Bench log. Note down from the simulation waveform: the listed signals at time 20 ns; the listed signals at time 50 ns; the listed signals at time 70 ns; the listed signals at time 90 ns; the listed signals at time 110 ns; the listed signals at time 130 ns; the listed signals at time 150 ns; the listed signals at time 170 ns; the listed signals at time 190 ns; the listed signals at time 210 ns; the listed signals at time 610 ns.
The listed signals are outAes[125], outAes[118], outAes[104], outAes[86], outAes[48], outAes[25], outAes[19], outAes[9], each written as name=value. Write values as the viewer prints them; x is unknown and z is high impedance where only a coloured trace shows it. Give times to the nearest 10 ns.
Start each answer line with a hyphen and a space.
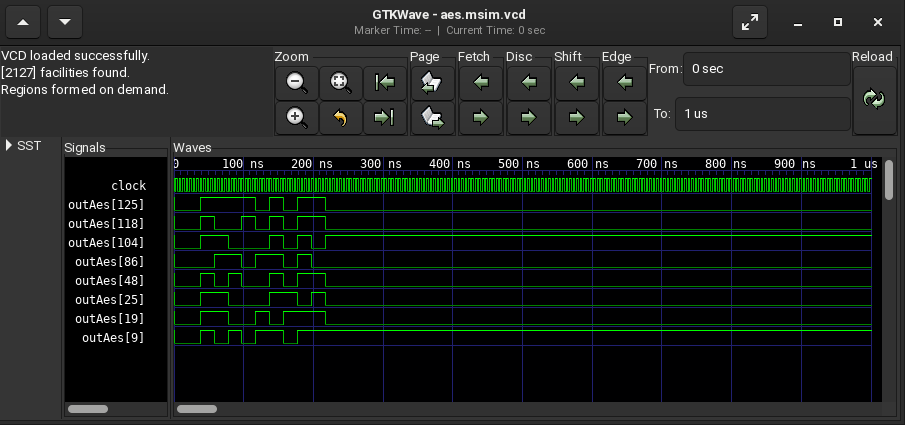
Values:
- outAes[125]=0, outAes[118]=0, outAes[104]=0, outAes[86]=0, outAes[48]=0, outAes[25]=0, outAes[19]=0, outAes[9]=0
- outAes[125]=1, outAes[118]=1, outAes[104]=1, outAes[86]=0, outAes[48]=1, outAes[25]=1, outAes[19]=1, outAes[9]=1
- outAes[125]=1, outAes[118]=0, outAes[104]=1, outAes[86]=1, outAes[48]=0, outAes[25]=1, outAes[19]=1, outAes[9]=0
- outAes[125]=1, outAes[118]=0, outAes[104]=0, outAes[86]=1, outAes[48]=1, outAes[25]=0, outAes[19]=0, outAes[9]=1
- outAes[125]=1, outAes[118]=1, outAes[104]=0, outAes[86]=0, outAes[48]=0, outAes[25]=0, outAes[19]=0, outAes[9]=0
- outAes[125]=0, outAes[118]=0, outAes[104]=0, outAes[86]=1, outAes[48]=0, outAes[25]=0, outAes[19]=1, outAes[9]=1
- outAes[125]=1, outAes[118]=1, outAes[104]=1, outAes[86]=1, outAes[48]=1, outAes[25]=1, outAes[19]=0, outAes[9]=1
- outAes[125]=0, outAes[118]=0, outAes[104]=0, outAes[86]=0, outAes[48]=0, outAes[25]=1, outAes[19]=1, outAes[9]=0
- outAes[125]=1, outAes[118]=1, outAes[104]=1, outAes[86]=1, outAes[48]=1, outAes[25]=0, outAes[19]=1, outAes[9]=1
- outAes[125]=1, outAes[118]=1, outAes[104]=0, outAes[86]=0, outAes[48]=1, outAes[25]=1, outAes[19]=1, outAes[9]=1
- outAes[125]=0, outAes[118]=0, outAes[104]=1, outAes[86]=0, outAes[48]=0, outAes[25]=0, outAes[19]=0, outAes[9]=1
